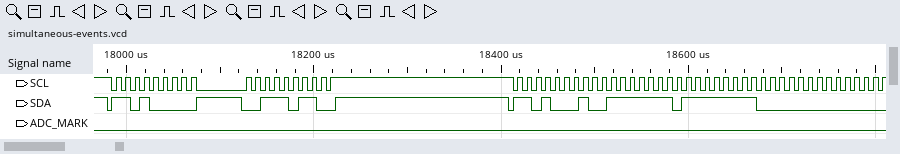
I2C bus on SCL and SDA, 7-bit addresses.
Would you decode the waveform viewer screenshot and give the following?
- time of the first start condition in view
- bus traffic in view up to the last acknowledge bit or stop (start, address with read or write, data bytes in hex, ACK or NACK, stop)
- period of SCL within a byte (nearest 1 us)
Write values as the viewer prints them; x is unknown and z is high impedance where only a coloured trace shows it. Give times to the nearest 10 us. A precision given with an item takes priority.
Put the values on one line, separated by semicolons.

17980 us; start, address 68 write ACK, 3B ACK, stop, start, address 68 read ACK, 7F ACK, FF ACK, 00 ACK; 10 us
